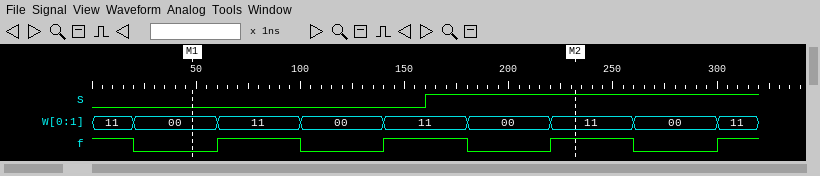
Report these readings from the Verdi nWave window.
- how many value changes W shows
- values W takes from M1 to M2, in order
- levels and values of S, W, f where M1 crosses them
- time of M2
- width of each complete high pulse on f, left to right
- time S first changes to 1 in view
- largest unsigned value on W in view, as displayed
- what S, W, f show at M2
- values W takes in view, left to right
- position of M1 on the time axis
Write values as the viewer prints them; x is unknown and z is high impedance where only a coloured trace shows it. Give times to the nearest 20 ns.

8
00, 11, 00, 11, 00, 11
S=0, W=00, f=0
240 ns
40 ns, 40 ns, 40 ns
160 ns
11
S=1, W=11, f=1
11, 00, 11, 00, 11, 00, 11, 00, 11
40 ns
